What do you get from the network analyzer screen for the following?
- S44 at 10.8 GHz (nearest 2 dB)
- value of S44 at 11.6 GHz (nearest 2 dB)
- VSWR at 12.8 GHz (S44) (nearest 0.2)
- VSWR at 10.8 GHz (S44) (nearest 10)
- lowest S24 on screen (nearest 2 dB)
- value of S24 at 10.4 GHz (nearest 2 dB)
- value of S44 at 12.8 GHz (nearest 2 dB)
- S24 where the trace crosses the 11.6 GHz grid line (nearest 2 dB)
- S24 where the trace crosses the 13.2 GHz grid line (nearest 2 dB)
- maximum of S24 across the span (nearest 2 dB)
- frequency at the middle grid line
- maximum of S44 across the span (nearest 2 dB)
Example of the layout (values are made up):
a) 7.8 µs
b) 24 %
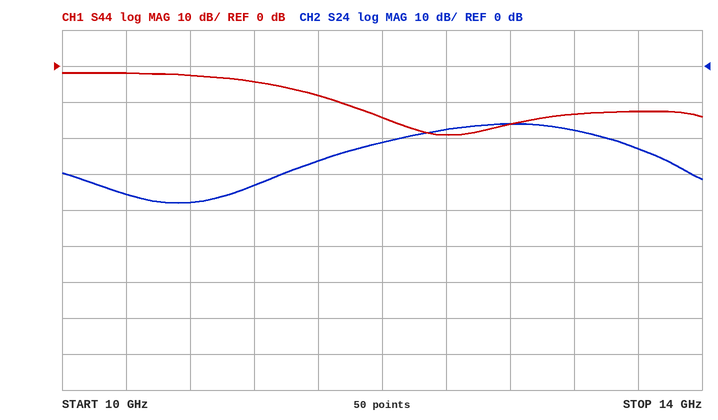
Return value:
a) -2 dB
b) -8 dB
c) 1.4
d) 10
e) -38 dB
f) -36 dB
g) -16 dB
h) -26 dB
i) -18 dB
j) -16 dB
k) 12 GHz
l) -2 dB
